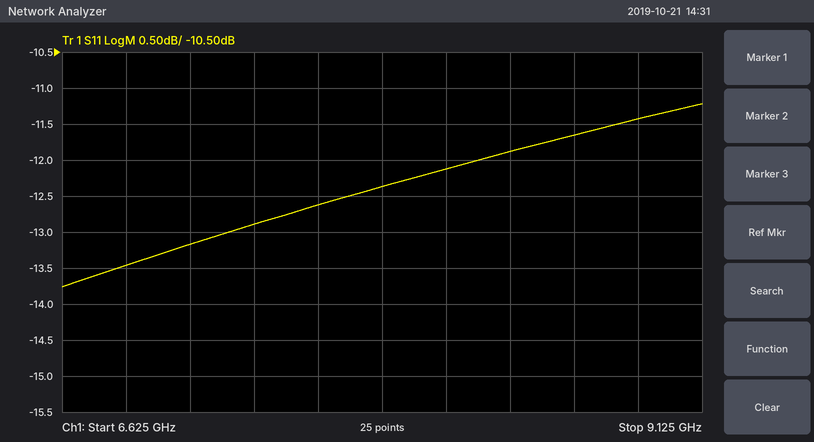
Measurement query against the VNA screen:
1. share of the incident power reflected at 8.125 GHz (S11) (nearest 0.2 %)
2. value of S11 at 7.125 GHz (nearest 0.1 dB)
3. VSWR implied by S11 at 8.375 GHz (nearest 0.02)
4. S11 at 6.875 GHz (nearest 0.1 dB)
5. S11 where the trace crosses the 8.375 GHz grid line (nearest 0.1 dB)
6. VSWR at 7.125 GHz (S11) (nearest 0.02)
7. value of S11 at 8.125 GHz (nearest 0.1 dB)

6.2 %
-13.2 dB
1.68
-13.5 dB
-11.9 dB
1.56
-12.1 dB
